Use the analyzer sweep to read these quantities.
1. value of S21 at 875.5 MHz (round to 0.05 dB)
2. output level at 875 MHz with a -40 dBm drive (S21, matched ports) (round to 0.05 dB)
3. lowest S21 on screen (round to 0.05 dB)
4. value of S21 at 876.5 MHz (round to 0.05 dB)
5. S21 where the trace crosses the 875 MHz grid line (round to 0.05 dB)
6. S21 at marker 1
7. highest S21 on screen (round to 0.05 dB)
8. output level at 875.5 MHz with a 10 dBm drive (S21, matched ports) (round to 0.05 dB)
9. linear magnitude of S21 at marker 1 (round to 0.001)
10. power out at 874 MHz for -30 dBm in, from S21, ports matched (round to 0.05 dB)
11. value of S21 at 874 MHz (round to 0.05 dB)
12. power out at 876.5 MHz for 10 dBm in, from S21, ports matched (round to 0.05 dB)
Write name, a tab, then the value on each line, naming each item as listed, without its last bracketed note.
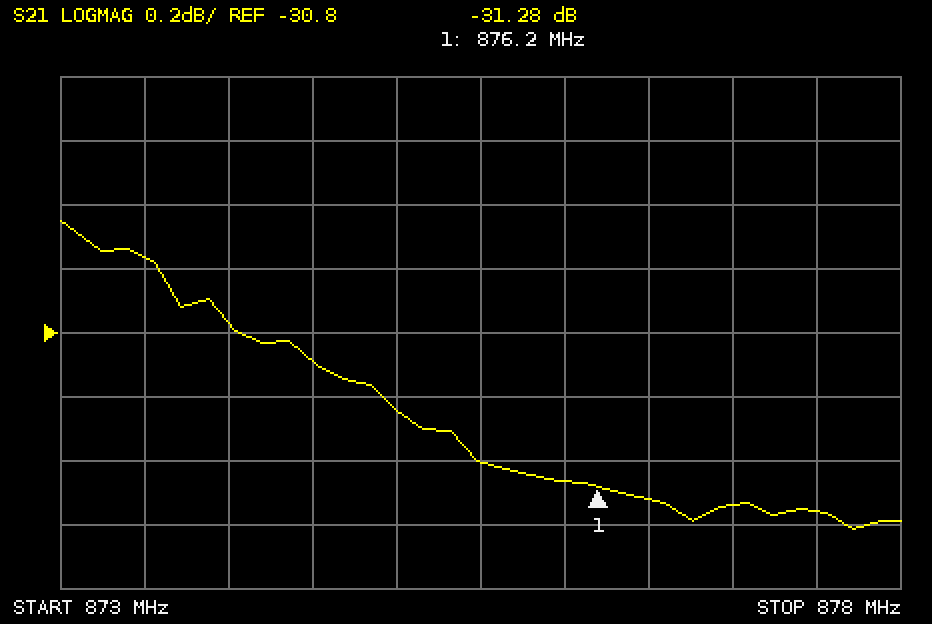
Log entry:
value of S21 at 875.5 MHz	-31.20 dB
output level at 875 MHz with a -40 dBm drive (S21, matched ports)	-71.05 dBm
lowest S21 on screen	-31.40 dB
value of S21 at 876.5 MHz	-31.30 dB
S21 where the trace crosses the 875 MHz grid line	-31.05 dB
S21 at marker 1	-31.28 dB
highest S21 on screen	-30.45 dB
output level at 875.5 MHz with a 10 dBm drive (S21, matched ports)	-21.20 dBm
linear magnitude of S21 at marker 1	0.027
power out at 874 MHz for -30 dBm in, from S21, ports matched	-60.75 dBm
value of S21 at 874 MHz	-30.75 dB
power out at 876.5 MHz for 10 dBm in, from S21, ports matched	-21.30 dBm
